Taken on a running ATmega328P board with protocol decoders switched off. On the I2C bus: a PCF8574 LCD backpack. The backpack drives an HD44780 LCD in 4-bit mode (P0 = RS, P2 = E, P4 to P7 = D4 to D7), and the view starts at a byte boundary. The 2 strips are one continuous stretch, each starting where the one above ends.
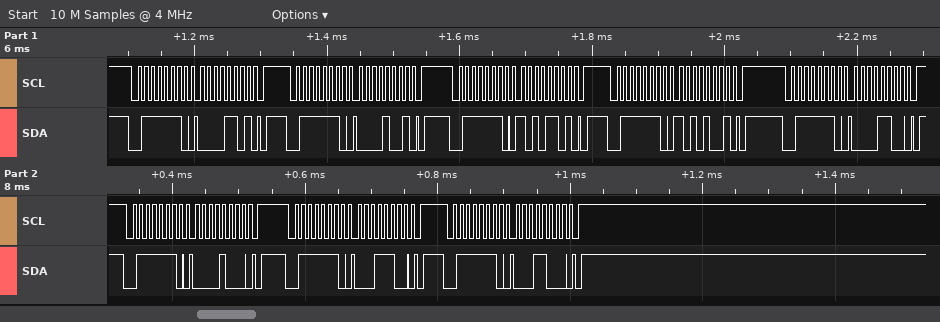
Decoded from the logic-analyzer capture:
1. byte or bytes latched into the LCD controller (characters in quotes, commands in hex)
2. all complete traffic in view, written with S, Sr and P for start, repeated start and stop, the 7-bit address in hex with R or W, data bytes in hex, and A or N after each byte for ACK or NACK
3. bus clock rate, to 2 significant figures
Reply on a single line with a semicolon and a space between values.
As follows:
data 0x0A 0x01; S 3FW A 0D A P S 3FW A 09 A P S 3FW A AD A P S 3FW A A9 A P S 3FW A 0C A P S 3FW A 08 A P S 3FW A 1C A P S 3FW A 18 A P; 100 kHz
